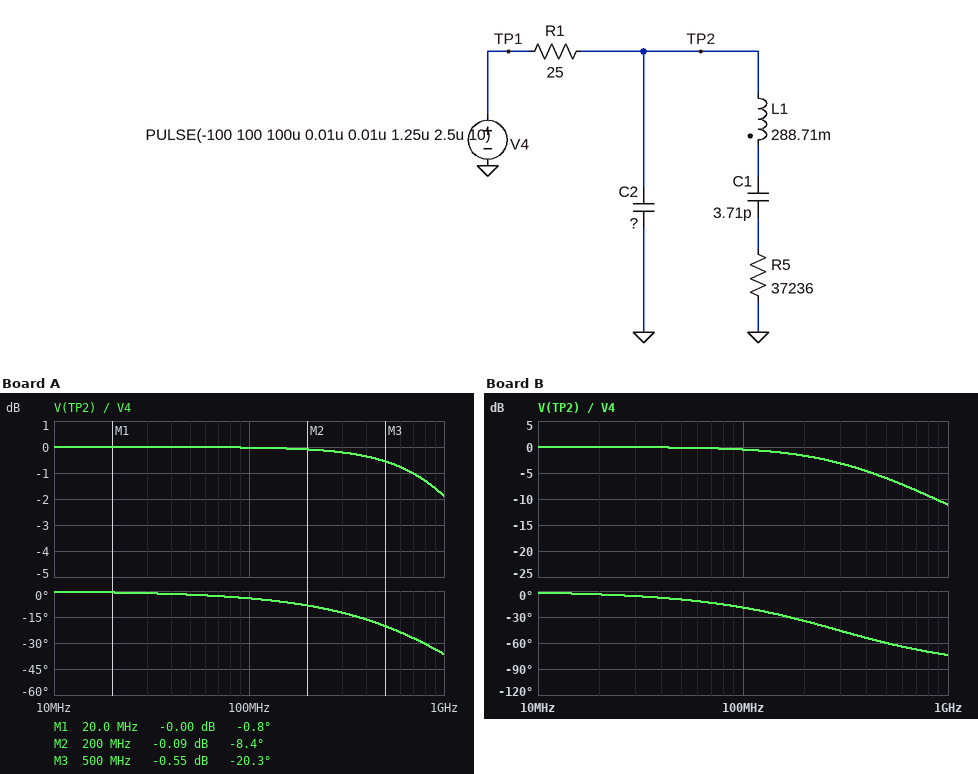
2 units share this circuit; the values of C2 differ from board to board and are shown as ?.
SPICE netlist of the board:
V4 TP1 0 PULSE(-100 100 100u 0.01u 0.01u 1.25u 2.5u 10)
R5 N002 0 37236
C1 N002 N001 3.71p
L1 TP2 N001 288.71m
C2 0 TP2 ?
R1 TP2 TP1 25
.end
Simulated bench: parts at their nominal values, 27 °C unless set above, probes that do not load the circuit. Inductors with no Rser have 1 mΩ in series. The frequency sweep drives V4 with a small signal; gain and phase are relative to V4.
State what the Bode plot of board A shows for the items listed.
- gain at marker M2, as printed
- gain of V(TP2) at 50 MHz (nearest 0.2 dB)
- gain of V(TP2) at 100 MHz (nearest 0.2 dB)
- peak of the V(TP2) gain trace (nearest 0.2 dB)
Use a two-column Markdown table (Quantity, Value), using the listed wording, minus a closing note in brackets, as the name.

| Quantity | Value |
|---|---|
| gain at marker M2, as printed | -0.09 dB |
| gain of V(TP2) at 50 MHz | 0 dB |
| gain of V(TP2) at 100 MHz | 0 dB |
| peak of the V(TP2) gain trace | 0 dB |
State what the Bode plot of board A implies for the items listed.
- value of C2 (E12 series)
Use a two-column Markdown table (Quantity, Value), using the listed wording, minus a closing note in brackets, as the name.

| Quantity | Value |
|---|---|
| value of C2 | 4.7 pF |
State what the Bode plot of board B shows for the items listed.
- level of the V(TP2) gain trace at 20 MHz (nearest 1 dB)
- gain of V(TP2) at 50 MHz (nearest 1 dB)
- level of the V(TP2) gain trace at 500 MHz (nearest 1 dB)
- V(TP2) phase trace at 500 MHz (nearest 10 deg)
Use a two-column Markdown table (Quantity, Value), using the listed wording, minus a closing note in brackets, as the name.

| Quantity | Value |
|---|---|
| level of the V(TP2) gain trace at 20 MHz | 0 dB |
| gain of V(TP2) at 50 MHz | 0 dB |
| level of the V(TP2) gain trace at 500 MHz | -6 dB |
| V(TP2) phase trace at 500 MHz | -60 deg |
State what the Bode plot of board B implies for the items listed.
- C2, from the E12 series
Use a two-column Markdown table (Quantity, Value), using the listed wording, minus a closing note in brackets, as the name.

| Quantity | Value |
|---|---|
| C2, from the E12 series | 22 pF |
